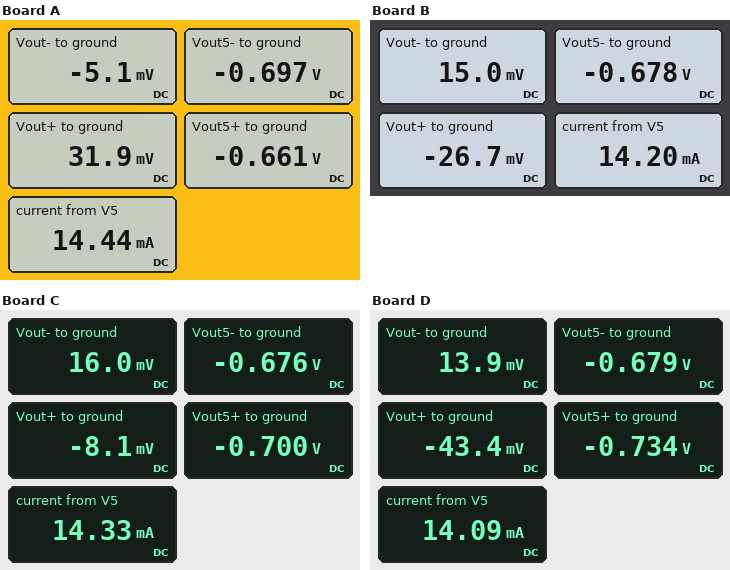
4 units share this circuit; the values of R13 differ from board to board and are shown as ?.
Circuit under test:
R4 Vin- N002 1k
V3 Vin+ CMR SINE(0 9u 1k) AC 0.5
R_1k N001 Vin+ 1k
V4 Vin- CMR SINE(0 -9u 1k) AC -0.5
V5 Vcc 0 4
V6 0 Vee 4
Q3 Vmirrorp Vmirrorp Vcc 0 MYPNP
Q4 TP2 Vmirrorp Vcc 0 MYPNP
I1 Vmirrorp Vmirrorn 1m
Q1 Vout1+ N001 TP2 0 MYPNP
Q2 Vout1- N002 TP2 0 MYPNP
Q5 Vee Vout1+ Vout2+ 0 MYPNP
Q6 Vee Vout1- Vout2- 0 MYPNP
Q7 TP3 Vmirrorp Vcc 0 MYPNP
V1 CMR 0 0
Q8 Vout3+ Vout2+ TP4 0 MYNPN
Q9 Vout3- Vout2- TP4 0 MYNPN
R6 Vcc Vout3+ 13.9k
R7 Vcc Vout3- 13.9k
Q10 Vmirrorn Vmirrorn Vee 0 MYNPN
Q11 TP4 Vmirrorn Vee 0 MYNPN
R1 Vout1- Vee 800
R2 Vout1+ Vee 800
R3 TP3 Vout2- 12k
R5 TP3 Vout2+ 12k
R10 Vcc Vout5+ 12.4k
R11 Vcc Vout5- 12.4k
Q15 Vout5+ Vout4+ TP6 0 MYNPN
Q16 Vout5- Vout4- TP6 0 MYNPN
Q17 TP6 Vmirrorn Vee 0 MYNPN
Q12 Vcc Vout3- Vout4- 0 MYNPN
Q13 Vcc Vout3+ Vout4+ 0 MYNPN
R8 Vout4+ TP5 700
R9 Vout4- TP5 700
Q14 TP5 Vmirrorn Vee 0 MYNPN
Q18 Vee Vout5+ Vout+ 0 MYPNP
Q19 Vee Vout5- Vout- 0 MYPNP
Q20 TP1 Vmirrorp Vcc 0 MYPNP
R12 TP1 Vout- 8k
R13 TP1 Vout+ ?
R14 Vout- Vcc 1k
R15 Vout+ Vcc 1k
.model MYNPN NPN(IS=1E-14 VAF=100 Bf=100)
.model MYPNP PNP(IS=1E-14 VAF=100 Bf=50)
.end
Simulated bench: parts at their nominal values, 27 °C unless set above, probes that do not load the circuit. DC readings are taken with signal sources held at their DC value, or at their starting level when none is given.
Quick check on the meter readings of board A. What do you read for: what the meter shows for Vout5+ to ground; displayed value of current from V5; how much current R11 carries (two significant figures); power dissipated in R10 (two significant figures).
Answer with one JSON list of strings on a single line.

["-0.661 V", "14.44 mA", "380 µA", "1.8 mW"]
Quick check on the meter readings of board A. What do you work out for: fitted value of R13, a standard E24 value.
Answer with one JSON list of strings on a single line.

["5.1 kΩ"]
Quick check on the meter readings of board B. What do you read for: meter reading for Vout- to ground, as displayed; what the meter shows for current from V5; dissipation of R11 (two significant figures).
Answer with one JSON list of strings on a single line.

["15.0 mV", "14.20 mA", "1.8 mW"]
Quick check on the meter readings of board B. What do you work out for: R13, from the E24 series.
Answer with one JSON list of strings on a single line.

["15 kΩ"]
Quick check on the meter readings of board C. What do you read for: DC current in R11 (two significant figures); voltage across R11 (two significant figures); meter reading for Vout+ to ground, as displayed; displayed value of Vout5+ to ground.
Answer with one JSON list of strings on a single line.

["380 µA", "4.7 V", "-8.1 mV", "-0.700 V"]
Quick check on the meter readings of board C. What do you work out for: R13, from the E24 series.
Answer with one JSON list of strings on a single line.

["11 kΩ"]
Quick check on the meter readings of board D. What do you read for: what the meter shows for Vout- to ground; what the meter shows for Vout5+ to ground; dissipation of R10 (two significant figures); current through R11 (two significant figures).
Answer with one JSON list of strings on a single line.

["13.9 mV", "-0.734 V", "1.8 mW", "380 µA"]
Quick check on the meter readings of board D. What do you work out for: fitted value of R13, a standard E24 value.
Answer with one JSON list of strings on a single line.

["22 kΩ"]
